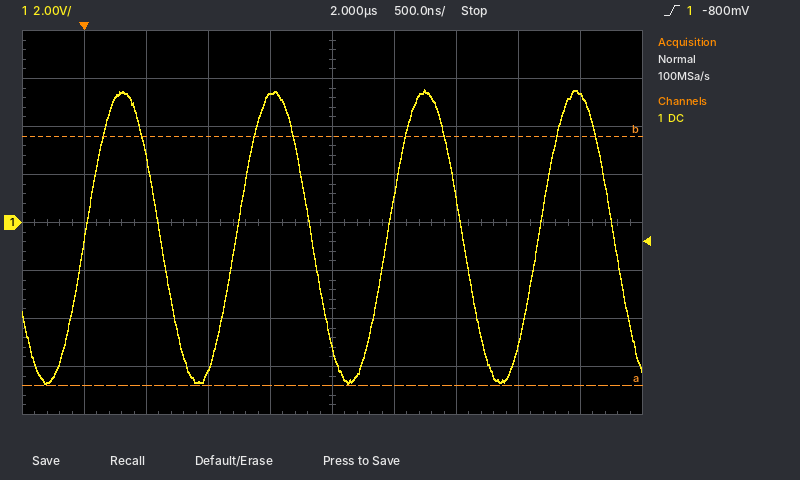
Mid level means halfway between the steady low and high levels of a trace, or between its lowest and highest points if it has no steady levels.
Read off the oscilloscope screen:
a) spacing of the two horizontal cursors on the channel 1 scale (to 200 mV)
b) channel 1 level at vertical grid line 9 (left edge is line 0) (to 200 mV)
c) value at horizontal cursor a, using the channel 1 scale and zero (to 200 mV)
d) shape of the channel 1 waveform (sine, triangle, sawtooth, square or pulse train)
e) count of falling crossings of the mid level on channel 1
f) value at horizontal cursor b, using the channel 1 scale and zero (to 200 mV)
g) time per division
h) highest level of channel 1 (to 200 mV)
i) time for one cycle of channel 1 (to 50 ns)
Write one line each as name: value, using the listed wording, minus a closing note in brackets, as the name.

spacing of the two horizontal cursors on the channel 1 scale: 10.4 V
channel 1 level at vertical grid line 9 (left edge is line 0): 5.4 V
value at horizontal cursor a, using the channel 1 scale and zero: -6.8 V
shape of the channel 1 waveform: sine
count of falling crossings of the mid level on channel 1: 4
value at horizontal cursor b, using the channel 1 scale and zero: 3.6 V
time per division: 500 ns
highest level of channel 1: 5.6 V
time for one cycle of channel 1: 1.20 µs
